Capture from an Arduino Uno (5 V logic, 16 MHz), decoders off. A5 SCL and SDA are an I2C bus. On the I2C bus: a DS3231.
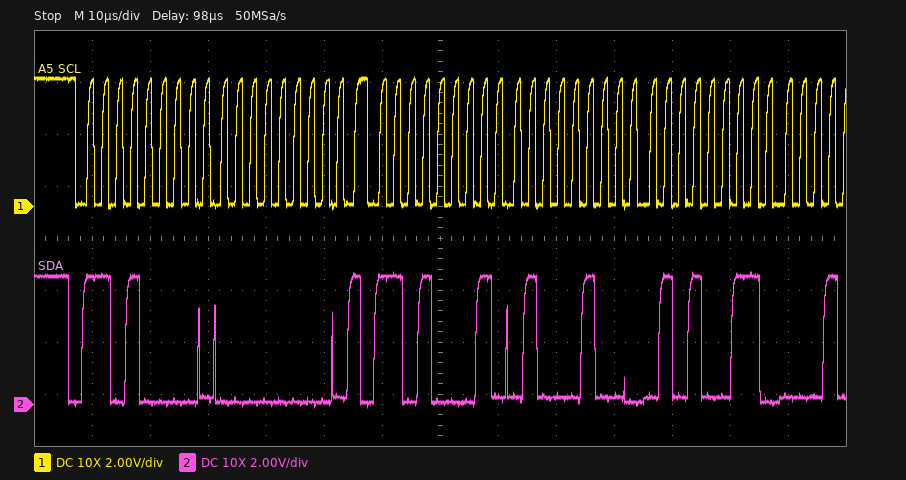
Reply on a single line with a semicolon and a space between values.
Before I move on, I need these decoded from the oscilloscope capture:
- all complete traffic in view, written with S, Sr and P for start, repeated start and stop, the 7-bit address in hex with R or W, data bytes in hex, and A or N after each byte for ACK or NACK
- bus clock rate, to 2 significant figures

S 68W A 00 A Sr 68R A 44 A 53 A; 400 kHz
